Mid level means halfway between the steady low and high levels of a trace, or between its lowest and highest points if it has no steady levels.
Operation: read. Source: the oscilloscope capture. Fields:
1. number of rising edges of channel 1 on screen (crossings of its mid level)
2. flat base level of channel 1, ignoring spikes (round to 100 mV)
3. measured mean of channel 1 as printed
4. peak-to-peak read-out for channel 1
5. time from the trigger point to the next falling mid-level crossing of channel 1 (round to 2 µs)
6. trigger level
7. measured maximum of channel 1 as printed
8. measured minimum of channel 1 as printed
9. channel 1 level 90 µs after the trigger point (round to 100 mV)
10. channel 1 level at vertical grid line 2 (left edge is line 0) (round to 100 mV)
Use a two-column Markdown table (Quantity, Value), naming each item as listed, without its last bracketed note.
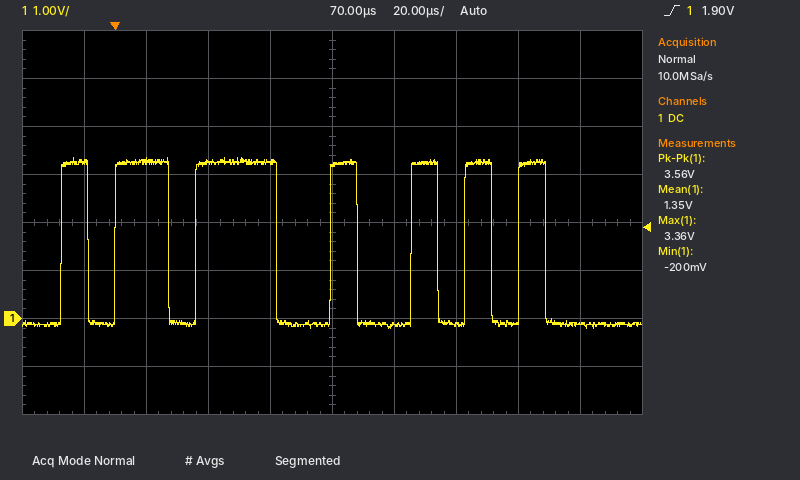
| Quantity | Value |
|---|---|
| number of rising edges of channel 1 on screen | 7 |
| flat base level of channel 1, ignoring spikes | -100 mV |
| measured mean of channel 1 as printed | 1.35 V |
| peak-to-peak read-out for channel 1 | 3.56 V |
| time from the trigger point to the next falling mid-level crossing of channel 1 | 18 µs |
| trigger level | 1.90 V |
| measured maximum of channel 1 as printed | 3.36 V |
| measured minimum of channel 1 as printed | -200 mV |
| channel 1 level 90 µs after the trigger point | -100 mV |
| channel 1 level at vertical grid line 2 (left edge is line 0) | 3.3 V |
